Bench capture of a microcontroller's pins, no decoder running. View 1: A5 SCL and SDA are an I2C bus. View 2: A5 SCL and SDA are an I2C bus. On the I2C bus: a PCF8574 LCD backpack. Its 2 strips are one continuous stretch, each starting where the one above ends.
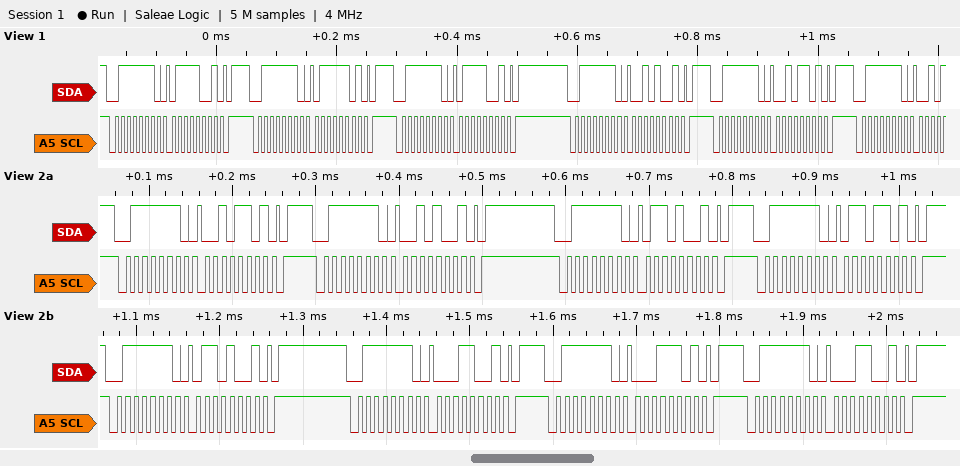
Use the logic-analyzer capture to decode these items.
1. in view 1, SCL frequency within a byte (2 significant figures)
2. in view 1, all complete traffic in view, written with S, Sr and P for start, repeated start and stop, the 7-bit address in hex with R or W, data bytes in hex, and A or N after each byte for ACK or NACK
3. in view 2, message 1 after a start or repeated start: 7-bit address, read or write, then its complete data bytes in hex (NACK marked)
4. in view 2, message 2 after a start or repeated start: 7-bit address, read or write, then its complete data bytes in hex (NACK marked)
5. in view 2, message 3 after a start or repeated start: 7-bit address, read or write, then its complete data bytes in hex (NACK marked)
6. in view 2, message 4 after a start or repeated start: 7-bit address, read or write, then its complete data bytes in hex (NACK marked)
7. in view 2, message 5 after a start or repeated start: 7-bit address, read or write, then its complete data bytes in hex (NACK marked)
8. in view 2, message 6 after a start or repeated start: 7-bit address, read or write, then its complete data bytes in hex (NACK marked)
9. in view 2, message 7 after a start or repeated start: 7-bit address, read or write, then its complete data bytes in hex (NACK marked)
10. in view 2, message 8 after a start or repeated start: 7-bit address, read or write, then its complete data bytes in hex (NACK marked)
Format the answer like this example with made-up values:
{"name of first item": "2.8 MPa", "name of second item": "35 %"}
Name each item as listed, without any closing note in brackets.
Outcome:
{"in view 1, SCL frequency within a byte": "100 kHz", "in view 1, all complete traffic in view, written with S, Sr and P for start, repeated start and stop, the 7-bit address in hex with R or W, data bytes in hex, and A or N after each byte for ACK or NACK": "S 3FW A 79 A P S 3FW A 7D A P S 3FW A 79 A P S 3FW A 29 A P S 3FW A 2D A P S 3FW A", "in view 2, message 1 after a start or repeated start: 7-bit address, read or write, then its complete data bytes in hex": "0x3F write: 2D", "in view 2, message 2 after a start or repeated start: 7-bit address, read or write, then its complete data bytes in hex": "0x3F write: 29", "in view 2, message 3 after a start or repeated start: 7-bit address, read or write, then its complete data bytes in hex": "0x3F write: 69", "in view 2, message 4 after a start or repeated start: 7-bit address, read or write, then its complete data bytes in hex": "0x3F write: 6D", "in view 2, message 5 after a start or repeated start: 7-bit address, read or write, then its complete data bytes in hex": "0x3F write: 69", "in view 2, message 6 after a start or repeated start: 7-bit address, read or write, then its complete data bytes in hex": "0x3F write: 19", "in view 2, message 7 after a start or repeated start: 7-bit address, read or write, then its complete data bytes in hex": "0x3F write: 1D", "in view 2, message 8 after a start or repeated start: 7-bit address, read or write, then its complete data bytes in hex": "0x3F write: 19"}
